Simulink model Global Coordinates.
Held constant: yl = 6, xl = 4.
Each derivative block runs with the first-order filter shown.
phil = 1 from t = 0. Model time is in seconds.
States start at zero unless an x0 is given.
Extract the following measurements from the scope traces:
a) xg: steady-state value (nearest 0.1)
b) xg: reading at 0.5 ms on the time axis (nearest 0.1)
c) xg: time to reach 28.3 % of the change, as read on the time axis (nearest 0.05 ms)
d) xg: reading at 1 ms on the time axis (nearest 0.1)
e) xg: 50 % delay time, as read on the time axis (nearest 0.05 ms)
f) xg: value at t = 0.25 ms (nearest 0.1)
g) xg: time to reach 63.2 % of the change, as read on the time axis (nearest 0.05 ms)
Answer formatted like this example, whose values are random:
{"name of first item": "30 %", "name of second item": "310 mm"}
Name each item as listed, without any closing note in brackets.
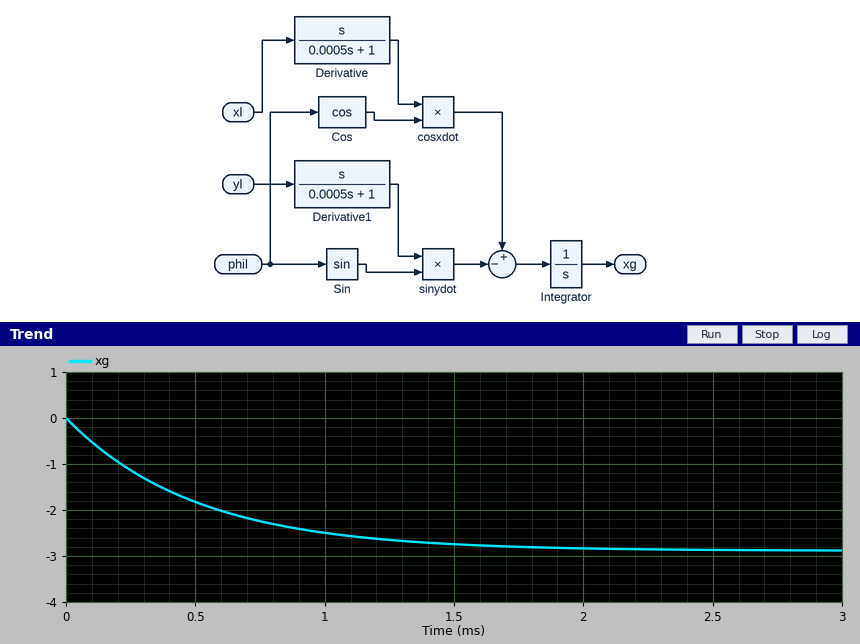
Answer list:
{"xg: steady-state value": "-2.9", "xg: reading at 0.5 ms on the time axis": "-1.8", "xg: time to reach 28.3 % of the change, as read on the time axis": "0.15 ms", "xg: reading at 1 ms on the time axis": "-2.5", "xg: 50 % delay time, as read on the time axis": "0.35 ms", "xg: value at t = 0.25 ms": "-1.1", "xg: time to reach 63.2 % of the change, as read on the time axis": "0.50 ms"}
